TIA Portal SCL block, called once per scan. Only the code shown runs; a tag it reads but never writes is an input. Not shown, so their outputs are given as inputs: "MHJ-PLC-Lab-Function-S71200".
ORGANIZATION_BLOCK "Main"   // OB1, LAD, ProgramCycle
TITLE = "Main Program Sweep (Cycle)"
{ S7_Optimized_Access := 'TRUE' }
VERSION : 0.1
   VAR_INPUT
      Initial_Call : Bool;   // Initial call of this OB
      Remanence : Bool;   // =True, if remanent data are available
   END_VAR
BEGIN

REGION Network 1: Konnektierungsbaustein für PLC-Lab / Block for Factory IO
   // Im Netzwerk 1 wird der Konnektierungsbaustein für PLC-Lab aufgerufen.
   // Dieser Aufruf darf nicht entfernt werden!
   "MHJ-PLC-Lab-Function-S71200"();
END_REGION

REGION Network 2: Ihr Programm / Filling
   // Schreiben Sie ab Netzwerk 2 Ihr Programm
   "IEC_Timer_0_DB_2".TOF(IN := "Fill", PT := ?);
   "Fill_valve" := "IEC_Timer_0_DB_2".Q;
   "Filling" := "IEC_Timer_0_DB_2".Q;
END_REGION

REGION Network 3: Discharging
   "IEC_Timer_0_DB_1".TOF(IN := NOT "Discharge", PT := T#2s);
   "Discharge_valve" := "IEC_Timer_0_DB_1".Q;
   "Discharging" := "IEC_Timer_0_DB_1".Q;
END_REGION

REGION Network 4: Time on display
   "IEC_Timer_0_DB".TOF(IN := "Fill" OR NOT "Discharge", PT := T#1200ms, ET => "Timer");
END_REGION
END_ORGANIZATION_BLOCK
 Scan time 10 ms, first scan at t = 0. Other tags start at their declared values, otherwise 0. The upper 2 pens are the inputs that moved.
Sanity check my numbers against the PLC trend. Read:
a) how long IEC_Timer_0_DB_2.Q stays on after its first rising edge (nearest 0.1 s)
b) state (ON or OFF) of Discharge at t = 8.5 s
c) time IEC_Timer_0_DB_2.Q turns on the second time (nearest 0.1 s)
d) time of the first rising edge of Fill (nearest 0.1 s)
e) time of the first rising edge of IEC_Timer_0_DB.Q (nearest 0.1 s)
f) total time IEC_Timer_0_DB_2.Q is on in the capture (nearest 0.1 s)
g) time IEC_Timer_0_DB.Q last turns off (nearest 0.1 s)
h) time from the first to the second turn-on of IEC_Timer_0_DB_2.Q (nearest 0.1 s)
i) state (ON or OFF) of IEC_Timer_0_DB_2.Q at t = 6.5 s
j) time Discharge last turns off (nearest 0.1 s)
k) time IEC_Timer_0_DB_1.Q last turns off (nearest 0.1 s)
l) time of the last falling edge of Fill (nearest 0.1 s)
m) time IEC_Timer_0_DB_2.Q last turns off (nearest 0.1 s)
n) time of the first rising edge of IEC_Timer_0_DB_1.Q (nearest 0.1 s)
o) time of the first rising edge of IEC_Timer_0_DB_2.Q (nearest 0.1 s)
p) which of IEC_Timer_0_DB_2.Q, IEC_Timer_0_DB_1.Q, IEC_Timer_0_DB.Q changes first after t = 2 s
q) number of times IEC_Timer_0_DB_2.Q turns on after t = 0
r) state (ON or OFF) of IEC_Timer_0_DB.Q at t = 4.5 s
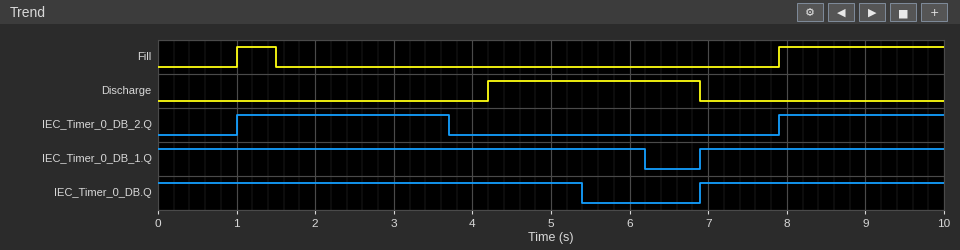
2.7 s
OFF
7.9 s
1.0 s
6.9 s
4.8 s
5.4 s
6.9 s
OFF
6.9 s
6.2 s
1.5 s
3.7 s
6.9 s
1.0 s
IEC_Timer_0_DB_2.Q
2
ON
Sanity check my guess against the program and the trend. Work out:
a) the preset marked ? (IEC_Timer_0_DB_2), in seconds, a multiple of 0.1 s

2.2 s
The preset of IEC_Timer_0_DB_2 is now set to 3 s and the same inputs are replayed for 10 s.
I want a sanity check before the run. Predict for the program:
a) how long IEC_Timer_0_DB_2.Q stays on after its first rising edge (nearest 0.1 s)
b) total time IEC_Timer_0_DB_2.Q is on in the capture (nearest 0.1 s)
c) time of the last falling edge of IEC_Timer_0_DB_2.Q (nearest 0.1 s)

3.5 s
5.6 s
4.5 s
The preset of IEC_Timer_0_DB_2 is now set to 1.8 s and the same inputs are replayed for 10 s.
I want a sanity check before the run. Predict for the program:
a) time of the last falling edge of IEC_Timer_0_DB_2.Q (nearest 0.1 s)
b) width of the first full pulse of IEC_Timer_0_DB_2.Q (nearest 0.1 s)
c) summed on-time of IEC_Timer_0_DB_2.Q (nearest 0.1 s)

3.3 s
2.3 s
4.4 s
